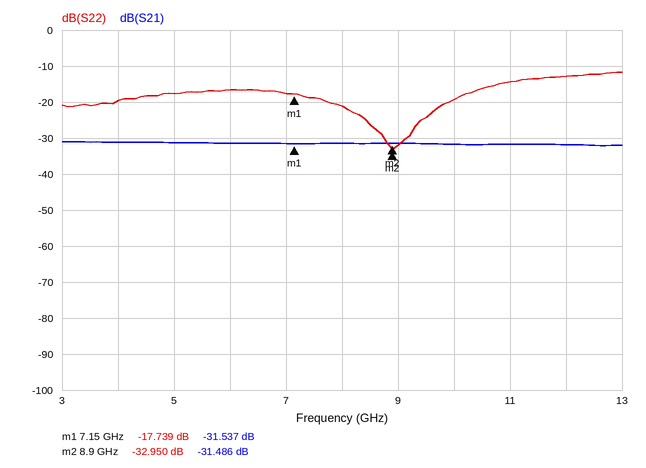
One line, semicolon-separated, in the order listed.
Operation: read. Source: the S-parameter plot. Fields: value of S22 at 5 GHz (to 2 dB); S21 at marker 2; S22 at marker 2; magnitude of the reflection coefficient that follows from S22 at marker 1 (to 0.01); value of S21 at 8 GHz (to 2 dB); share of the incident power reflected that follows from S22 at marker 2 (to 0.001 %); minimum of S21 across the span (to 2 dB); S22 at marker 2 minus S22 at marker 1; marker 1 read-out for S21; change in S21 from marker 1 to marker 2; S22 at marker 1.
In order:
-18 dB; -31.486 dB; -32.950 dB; 0.13; -32 dB; 0.051 %; -32 dB; -15.211 dB; -31.537 dB; 0.051 dB; -17.739 dB
